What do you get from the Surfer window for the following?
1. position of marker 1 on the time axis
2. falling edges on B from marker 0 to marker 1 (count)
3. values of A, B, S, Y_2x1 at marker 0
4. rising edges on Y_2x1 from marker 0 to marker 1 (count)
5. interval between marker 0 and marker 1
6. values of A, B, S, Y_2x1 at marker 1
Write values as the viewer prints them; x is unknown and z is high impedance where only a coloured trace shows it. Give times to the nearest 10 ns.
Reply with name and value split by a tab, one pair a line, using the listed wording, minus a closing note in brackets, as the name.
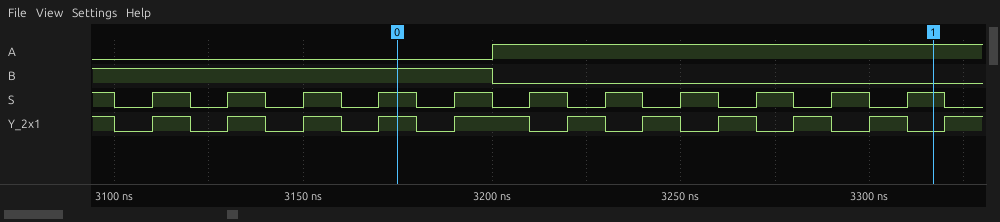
position of marker 1 on the time axis	3320 ns
falling edges on B from marker 0 to marker 1	1
values of A, B, S, Y_2x1 at marker 0	A=0, B=1, S=1, Y_2x1=1
rising edges on Y_2x1 from marker 0 to marker 1	6
interval between marker 0 and marker 1	140 ns
values of A, B, S, Y_2x1 at marker 1	A=1, B=0, S=1, Y_2x1=0
